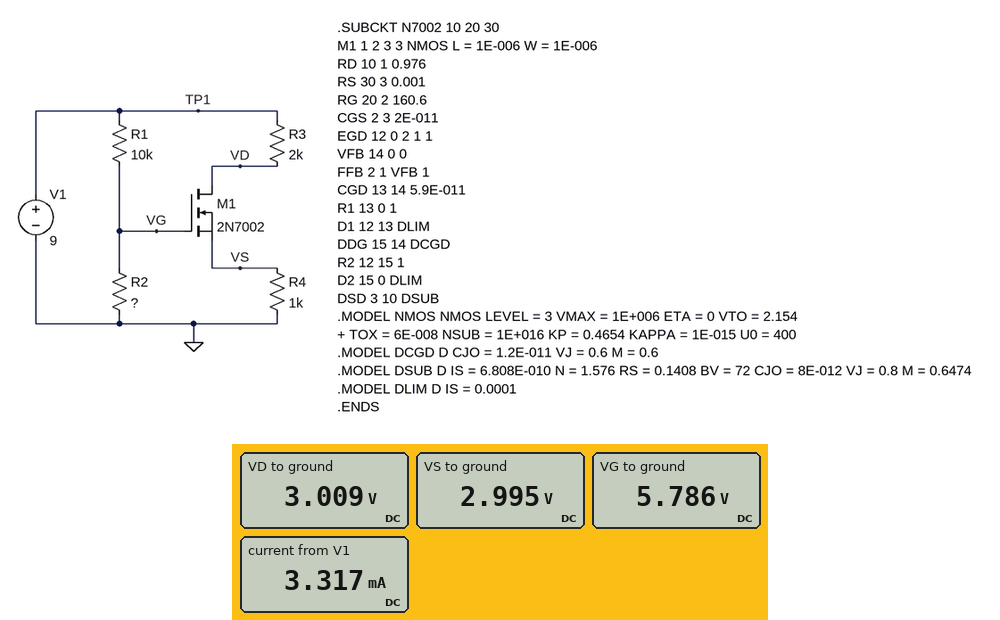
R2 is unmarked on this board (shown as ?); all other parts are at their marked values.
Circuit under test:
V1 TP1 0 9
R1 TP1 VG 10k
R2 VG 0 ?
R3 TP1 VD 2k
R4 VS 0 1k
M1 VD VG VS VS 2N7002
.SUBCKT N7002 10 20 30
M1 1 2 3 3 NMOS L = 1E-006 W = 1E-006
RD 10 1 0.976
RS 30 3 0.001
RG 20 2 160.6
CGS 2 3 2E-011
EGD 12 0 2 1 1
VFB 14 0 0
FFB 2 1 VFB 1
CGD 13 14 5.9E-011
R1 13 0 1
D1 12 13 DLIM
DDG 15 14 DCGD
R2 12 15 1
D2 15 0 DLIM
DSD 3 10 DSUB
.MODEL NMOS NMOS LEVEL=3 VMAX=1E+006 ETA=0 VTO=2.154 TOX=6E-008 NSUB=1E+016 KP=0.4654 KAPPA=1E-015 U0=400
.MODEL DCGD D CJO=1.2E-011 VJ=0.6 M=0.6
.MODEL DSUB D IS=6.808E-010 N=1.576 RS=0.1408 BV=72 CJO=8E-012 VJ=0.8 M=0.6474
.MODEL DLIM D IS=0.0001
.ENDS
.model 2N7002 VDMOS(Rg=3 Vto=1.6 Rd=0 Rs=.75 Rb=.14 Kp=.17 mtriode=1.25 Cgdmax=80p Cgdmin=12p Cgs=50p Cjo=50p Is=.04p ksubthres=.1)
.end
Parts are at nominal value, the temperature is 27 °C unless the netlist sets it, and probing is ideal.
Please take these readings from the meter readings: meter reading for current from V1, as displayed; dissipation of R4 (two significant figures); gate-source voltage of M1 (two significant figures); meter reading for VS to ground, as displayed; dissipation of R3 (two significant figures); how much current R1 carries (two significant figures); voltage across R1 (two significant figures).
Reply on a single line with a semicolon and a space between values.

3.317 mA; 9.0 mW; 2.8 V; 2.995 V; 18 mW; 320 µA; 3.2 V
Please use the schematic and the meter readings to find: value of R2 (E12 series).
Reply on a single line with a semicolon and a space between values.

18 kΩ
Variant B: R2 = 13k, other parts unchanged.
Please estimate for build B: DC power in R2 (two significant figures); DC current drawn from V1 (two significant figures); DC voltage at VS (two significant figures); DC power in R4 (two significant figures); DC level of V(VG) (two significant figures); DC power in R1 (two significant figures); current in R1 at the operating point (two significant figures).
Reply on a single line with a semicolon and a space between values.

2.0 mW; 3.4 mA; 3.0 V; 8.9 mW; 5.1 V; 1.5 mW; 390 µA
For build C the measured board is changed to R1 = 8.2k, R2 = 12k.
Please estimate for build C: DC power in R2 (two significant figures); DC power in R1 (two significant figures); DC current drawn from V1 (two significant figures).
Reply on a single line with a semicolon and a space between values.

2.4 mW; 1.6 mW; 3.4 mA
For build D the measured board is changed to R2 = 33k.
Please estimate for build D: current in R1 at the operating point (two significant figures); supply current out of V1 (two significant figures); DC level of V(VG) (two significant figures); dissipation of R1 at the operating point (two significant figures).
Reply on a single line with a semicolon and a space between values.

210 µA; 3.2 mA; 6.9 V; 440 µW
